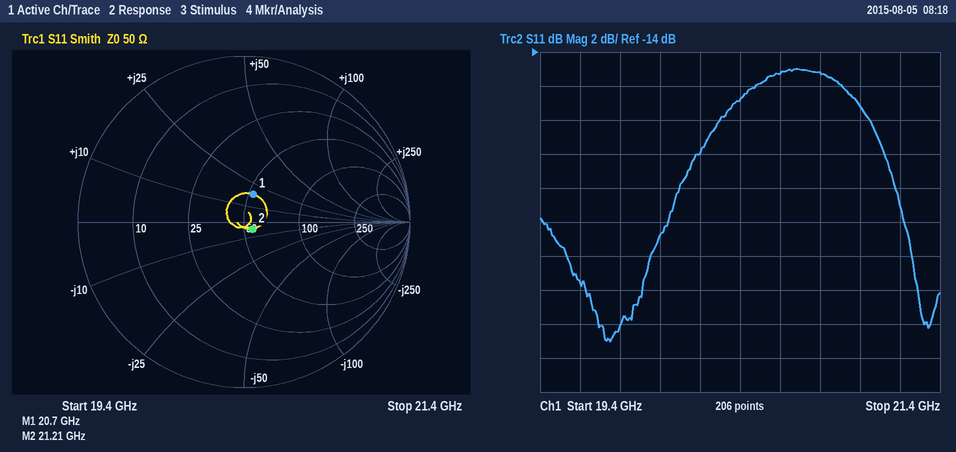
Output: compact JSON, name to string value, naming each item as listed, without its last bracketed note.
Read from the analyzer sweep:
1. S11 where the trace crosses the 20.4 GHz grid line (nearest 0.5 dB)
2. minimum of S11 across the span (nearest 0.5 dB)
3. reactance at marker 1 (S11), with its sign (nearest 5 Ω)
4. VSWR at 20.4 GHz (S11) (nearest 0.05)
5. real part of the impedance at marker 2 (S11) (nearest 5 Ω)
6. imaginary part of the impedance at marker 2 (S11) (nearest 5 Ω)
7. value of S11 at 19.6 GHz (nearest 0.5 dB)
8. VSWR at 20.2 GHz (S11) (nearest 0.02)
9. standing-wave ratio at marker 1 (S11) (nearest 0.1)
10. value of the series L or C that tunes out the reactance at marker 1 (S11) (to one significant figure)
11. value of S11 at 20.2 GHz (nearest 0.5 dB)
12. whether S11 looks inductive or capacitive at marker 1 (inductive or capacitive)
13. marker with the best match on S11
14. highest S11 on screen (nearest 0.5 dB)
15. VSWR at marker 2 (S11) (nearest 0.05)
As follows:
{"S11 where the trace crosses the 20.4 GHz grid line": "-17.0 dB", "minimum of S11 across the span": "-31.0 dB", "reactance at marker 1 (S11), with its sign": "+20 Ω", "VSWR at 20.4 GHz (S11)": "1.35", "real part of the impedance at marker 2 (S11)": "55 Ω", "imaginary part of the impedance at marker 2 (S11)": "-5 Ω", "value of S11 at 19.6 GHz": "-27.5 dB", "VSWR at 20.2 GHz (S11)": "1.22", "standing-wave ratio at marker 1 (S11)": "1.4", "value of the series L or C that tunes out the reactance at marker 1 (S11)": "400 fF", "value of S11 at 20.2 GHz": "-20.0 dB", "whether S11 looks inductive or capacitive at marker 1": "inductive", "marker with the best match on S11": "marker 2", "highest S11 on screen": "-15.0 dB", "VSWR at marker 2 (S11)": "1.15"}
